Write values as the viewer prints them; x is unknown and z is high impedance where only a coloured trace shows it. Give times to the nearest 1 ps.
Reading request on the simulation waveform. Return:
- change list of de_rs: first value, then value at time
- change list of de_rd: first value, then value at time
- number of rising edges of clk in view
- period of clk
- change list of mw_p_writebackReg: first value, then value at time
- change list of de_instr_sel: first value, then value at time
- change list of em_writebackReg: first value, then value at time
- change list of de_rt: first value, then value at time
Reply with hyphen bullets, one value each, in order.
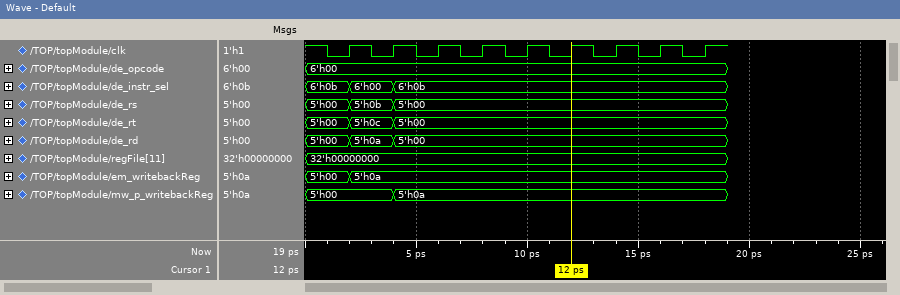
- 5'h00, 5'h0b at 2 ps, 5'h00 at 4 ps
- 5'h00, 5'h0a at 2 ps, 5'h00 at 4 ps
- 9
- 2 ps
- 5'h00, 5'h0a at 4 ps
- 6'h0b, 6'h00 at 2 ps, 6'h0b at 4 ps
- 5'h00, 5'h0a at 2 ps
- 5'h00, 5'h0c at 2 ps, 5'h00 at 4 ps
